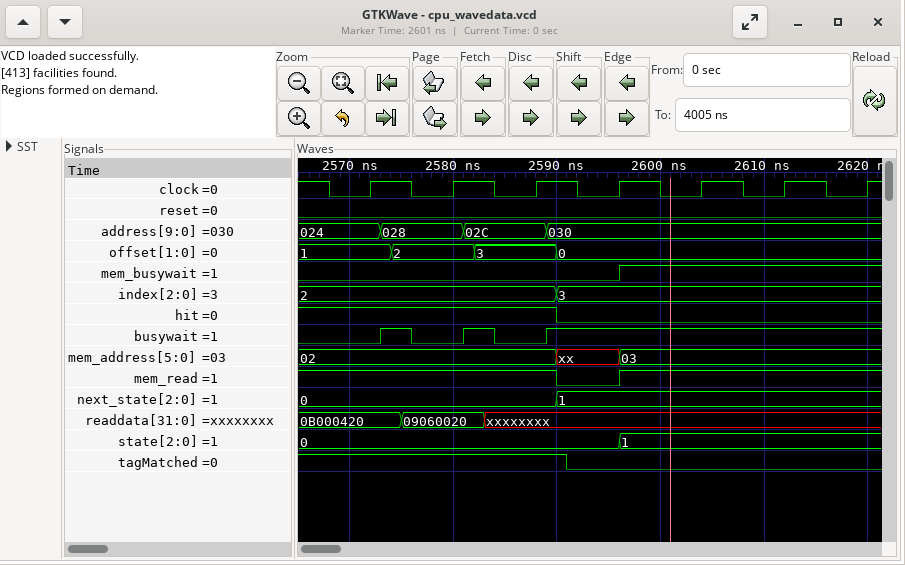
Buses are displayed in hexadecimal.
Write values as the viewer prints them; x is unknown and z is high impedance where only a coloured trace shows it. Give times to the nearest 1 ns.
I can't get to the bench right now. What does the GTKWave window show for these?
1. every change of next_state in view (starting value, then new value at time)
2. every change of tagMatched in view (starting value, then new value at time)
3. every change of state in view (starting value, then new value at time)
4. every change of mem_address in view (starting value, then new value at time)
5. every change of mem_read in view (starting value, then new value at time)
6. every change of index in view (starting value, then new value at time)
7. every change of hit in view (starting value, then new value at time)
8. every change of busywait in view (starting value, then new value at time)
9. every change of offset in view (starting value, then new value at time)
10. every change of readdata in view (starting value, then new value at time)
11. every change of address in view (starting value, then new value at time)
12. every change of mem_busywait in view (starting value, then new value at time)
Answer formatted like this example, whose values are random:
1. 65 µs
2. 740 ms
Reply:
1. 0, 1 at 2590 ns
2. 1, 0 at 2591 ns
3. 0, 1 at 2596 ns
4. 02, xx at 2590 ns, 03 at 2596 ns
5. 1, 0 at 2590 ns, 1 at 2596 ns
6. 2, 3 at 2590 ns
7. 1, 0 at 2590 ns
8. 0, 1 at 2573 ns, 0 at 2576 ns, 1 at 2581 ns, 0 at 2584 ns, 1 at 2589 ns
9. 1, 2 at 2574 ns, 3 at 2582 ns, 0 at 2590 ns
10. 0B000420, 09060020 at 2575 ns, xxxxxxxx at 2583 ns
11. 024, 028 at 2573 ns, 02C at 2581 ns, 030 at 2589 ns
12. 0, 1 at 2596 ns
